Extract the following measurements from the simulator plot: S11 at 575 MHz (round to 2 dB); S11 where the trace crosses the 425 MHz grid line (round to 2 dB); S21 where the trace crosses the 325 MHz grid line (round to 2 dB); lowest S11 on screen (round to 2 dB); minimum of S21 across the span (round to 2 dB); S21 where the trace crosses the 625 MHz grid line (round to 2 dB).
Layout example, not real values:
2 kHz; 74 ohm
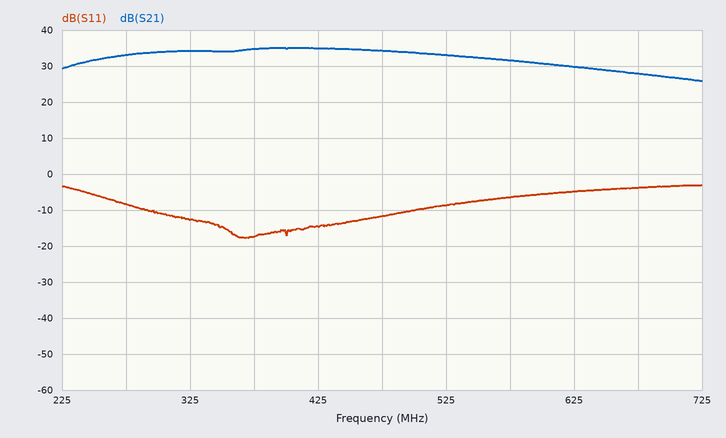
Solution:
-6 dB; -14 dB; 34 dB; -18 dB; 26 dB; 30 dB
